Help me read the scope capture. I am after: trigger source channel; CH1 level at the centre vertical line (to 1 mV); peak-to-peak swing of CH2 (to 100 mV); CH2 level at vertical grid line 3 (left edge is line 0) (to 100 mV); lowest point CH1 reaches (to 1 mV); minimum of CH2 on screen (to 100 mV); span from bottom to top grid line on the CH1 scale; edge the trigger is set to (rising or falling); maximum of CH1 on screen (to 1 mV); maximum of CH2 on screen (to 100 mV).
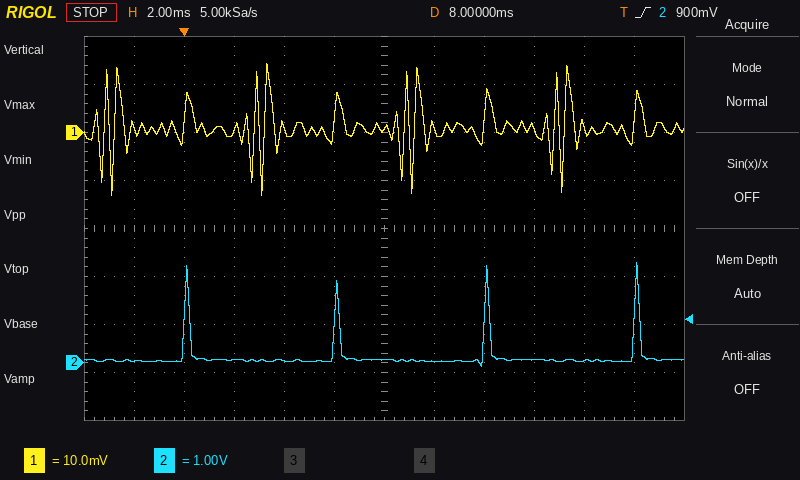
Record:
CH2
1 mV
2.2 V
100 mV
-13 mV
-100 mV
80 mV
rising
14 mV
2.1 V
